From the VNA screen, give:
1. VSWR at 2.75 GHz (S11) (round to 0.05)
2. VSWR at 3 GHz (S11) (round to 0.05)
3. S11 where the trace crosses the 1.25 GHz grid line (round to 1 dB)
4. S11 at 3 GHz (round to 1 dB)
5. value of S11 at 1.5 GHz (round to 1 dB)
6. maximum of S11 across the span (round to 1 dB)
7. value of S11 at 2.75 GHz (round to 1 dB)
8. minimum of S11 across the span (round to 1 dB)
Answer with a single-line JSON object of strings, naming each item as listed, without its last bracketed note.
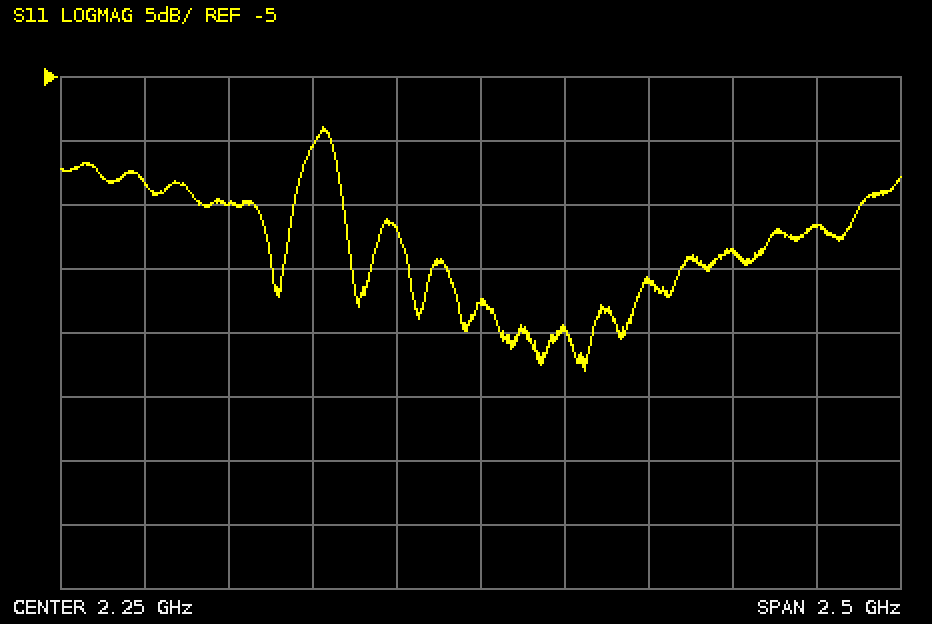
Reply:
{"VSWR at 2.75 GHz (S11)": "1.20", "VSWR at 3 GHz (S11)": "1.25", "S11 where the trace crosses the 1.25 GHz grid line": "-13 dB", "S11 at 3 GHz": "-19 dB", "value of S11 at 1.5 GHz": "-15 dB", "maximum of S11 across the span": "-9 dB", "value of S11 at 2.75 GHz": "-21 dB", "minimum of S11 across the span": "-28 dB"}
